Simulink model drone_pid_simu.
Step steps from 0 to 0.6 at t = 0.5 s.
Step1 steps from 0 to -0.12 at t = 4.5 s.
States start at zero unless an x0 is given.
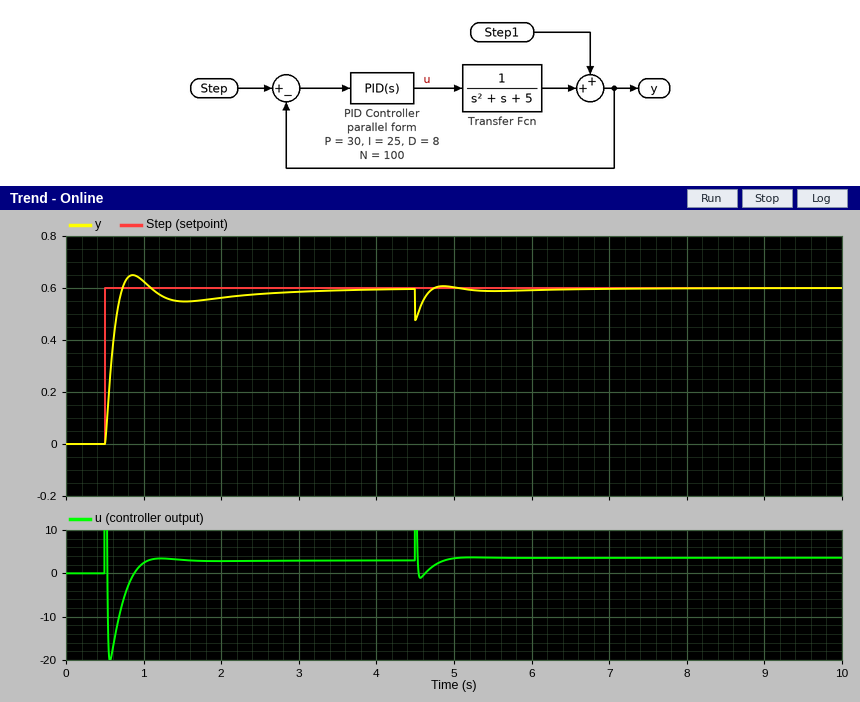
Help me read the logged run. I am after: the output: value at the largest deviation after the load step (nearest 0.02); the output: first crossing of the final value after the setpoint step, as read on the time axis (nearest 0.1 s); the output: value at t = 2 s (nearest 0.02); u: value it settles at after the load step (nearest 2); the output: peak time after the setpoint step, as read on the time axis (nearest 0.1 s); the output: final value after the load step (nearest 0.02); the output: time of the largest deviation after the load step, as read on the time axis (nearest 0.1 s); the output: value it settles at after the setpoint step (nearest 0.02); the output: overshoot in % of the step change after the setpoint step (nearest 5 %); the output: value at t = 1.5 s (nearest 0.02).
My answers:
0.48
0.7 s
0.56
4
0.9 s
0.60
4.5 s
0.60
10 %
0.54
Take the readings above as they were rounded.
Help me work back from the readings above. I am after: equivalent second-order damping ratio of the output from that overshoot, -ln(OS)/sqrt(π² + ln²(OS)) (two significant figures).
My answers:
0.59
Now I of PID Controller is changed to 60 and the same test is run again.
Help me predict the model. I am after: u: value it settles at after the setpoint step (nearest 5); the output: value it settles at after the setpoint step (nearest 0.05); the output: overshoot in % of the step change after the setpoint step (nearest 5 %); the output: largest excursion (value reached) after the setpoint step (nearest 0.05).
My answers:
5
0.60
15 %
0.70
